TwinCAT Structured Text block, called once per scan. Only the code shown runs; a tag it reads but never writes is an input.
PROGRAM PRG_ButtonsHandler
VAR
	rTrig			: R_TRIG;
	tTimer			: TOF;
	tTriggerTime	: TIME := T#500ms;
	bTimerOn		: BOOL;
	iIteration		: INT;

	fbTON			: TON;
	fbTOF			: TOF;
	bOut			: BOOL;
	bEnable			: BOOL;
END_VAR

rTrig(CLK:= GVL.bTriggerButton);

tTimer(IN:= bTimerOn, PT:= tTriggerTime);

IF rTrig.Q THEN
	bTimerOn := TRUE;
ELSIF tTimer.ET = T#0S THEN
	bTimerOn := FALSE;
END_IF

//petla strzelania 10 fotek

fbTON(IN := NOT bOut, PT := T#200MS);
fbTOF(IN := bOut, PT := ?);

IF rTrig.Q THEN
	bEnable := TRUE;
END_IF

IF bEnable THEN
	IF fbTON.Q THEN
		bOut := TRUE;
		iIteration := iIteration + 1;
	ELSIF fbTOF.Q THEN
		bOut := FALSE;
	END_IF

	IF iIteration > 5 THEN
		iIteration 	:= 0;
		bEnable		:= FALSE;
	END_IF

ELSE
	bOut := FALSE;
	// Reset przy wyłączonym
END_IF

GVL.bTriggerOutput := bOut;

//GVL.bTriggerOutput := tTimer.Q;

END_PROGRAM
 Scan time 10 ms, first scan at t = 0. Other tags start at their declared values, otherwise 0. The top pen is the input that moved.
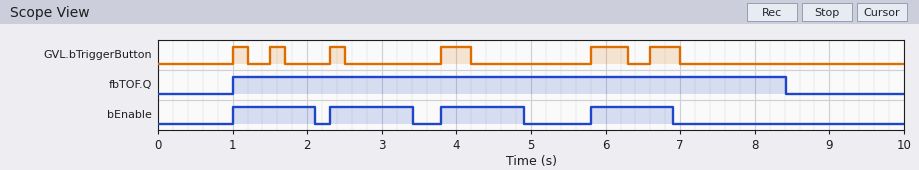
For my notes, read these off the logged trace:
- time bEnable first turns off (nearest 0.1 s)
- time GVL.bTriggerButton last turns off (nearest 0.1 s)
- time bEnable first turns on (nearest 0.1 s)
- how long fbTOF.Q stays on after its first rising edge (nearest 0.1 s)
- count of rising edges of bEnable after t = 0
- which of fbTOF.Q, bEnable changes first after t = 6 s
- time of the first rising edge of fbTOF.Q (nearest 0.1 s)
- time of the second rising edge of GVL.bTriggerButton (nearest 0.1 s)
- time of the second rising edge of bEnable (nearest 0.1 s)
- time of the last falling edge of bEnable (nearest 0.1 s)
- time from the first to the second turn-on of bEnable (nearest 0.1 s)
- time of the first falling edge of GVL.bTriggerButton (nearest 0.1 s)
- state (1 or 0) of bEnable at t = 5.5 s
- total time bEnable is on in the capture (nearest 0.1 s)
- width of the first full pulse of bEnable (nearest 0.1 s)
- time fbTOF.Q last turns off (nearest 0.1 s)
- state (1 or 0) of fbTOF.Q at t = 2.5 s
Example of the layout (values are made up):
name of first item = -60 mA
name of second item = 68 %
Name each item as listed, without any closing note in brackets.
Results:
time bEnable first turns off = 2.1 s
time GVL.bTriggerButton last turns off = 7.0 s
time bEnable first turns on = 1.0 s
how long fbTOF.Q stays on after its first rising edge = 7.4 s
count of rising edges of bEnable after t = 0 = 4
which of fbTOF.Q, bEnable changes first after t = 6 s = bEnable
time of the first rising edge of fbTOF.Q = 1.0 s
time of the second rising edge of GVL.bTriggerButton = 1.5 s
time of the second rising edge of bEnable = 2.3 s
time of the last falling edge of bEnable = 6.9 s
time from the first to the second turn-on of bEnable = 1.3 s
time of the first falling edge of GVL.bTriggerButton = 1.2 s
state (1 or 0) of bEnable at t = 5.5 s = 0
total time bEnable is on in the capture = 4.4 s
width of the first full pulse of bEnable = 1.1 s
time fbTOF.Q last turns off = 8.4 s
state (1 or 0) of fbTOF.Q at t = 2.5 s = 1
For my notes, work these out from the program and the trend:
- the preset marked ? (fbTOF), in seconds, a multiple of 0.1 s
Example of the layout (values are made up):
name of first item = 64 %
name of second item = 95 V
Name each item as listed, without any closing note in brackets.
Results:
the preset marked ? (fbTOF), in seconds, a multiple of 0.1 s = 1.5 s
